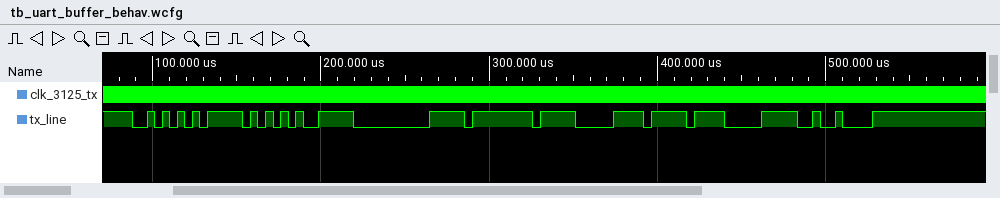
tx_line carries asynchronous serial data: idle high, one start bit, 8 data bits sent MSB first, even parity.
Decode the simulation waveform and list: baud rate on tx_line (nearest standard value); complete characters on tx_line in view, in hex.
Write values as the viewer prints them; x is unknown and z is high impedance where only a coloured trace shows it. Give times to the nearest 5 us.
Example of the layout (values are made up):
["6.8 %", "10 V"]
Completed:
["230400 baud", "55, AA, 00, FF, 0F, F0, 48"]
